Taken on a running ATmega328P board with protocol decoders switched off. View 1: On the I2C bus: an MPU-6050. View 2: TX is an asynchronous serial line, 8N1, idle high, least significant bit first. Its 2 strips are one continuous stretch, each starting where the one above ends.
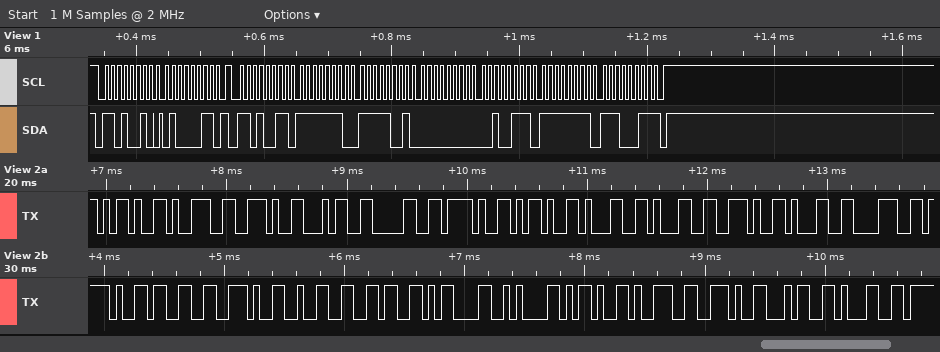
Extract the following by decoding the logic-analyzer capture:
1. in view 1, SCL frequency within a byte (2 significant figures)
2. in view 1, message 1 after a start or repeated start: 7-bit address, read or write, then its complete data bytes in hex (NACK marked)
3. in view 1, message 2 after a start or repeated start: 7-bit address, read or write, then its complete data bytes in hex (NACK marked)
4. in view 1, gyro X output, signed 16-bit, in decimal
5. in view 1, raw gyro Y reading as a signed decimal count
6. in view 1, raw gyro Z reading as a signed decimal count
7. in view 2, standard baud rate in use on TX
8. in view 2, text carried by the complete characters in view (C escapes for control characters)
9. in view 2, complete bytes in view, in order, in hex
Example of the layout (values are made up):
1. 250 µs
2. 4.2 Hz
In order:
1. 100 kHz
2. 0x69 write: 43
3. 0x69 read: FE F9 00 27 FF E3 NACK
4. -263
5. 39
6. -29
7. 19200 baud
8. "-9.40/-11.18/3.26\r\n-9.41"
9. 2D 39 2E 34 30 2F 2D 31 31 2E 31 38 2F 33 2E 32 36 0D 0A 2D 39 2E 34 31
